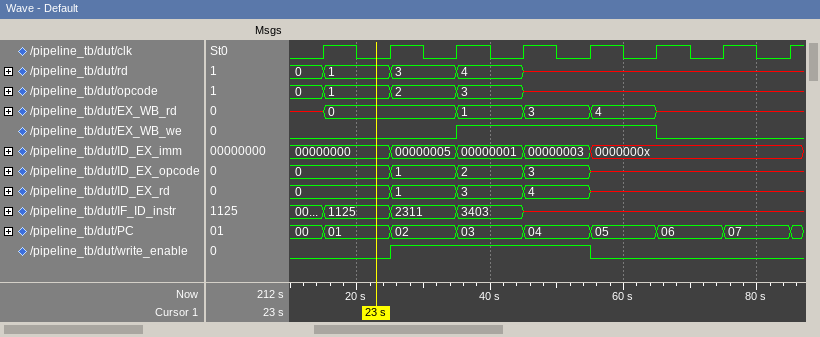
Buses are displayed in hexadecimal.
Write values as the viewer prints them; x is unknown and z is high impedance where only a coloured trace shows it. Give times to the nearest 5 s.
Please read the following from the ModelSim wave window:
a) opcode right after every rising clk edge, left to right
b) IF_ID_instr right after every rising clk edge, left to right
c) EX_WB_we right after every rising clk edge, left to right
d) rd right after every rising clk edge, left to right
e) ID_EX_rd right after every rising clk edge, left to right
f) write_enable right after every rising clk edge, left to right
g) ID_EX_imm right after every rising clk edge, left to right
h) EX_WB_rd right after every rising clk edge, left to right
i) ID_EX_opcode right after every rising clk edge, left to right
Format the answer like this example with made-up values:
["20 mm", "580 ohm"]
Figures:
["1, 2, 3, x, x, x, x, x", "1125, 2311, 3403, x, x, x, x, x", "0 0 1 1 1 0 0 0", "1, 3, 4, x, x, x, x, x", "0, 1, 3, 4, x, x, x, x", "0 1 1 1 0 0 0 0", "00000000, 00000005, 00000001, 00000003, 0000000x, 0000000x, 0000000x, 0000000x", "0, 0, 1, 3, 4, x, x, x", "0, 1, 2, 3, x, x, x, x"]
